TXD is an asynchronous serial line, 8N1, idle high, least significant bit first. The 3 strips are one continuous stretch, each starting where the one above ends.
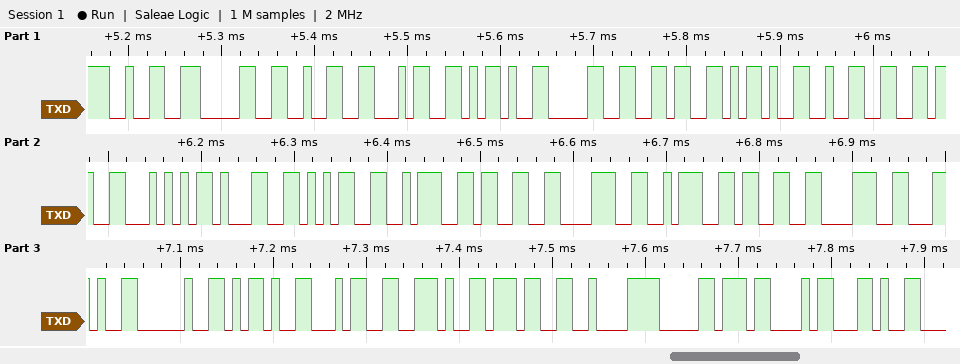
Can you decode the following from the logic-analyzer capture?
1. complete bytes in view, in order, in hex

32 30 32 34 2D 30 36 2D 32 36 54 31 35 3A 33 38 3A 33 38 2C 20 2D 34 2E 37 C2 B0 43 2C
